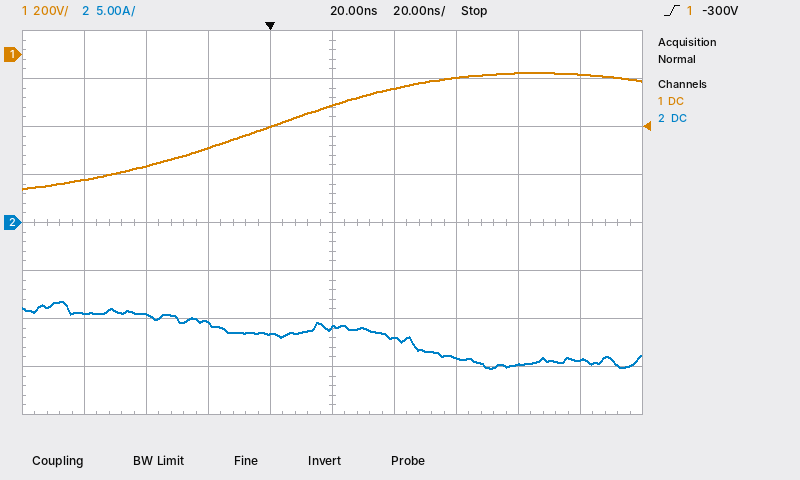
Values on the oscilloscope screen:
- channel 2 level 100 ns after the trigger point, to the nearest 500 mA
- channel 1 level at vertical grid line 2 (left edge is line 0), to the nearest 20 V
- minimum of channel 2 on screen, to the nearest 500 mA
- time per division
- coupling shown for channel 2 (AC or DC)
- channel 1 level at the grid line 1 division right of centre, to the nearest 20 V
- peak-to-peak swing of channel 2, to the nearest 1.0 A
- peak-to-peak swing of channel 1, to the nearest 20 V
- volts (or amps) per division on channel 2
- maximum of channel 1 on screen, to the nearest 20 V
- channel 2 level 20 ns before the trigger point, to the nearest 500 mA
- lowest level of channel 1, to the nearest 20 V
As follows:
-14.5 A
-460 V
-15.0 A
20 ns
DC
-140 V
7.0 A
480 V
5 A
-80 V
-10.5 A
-560 V
